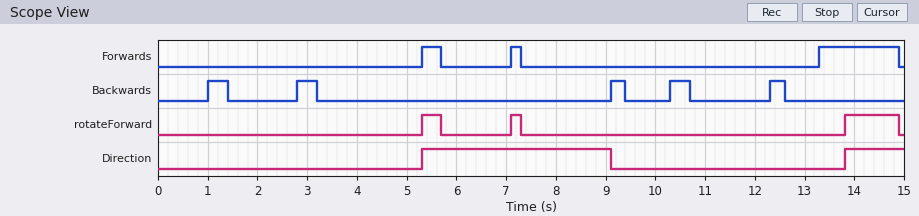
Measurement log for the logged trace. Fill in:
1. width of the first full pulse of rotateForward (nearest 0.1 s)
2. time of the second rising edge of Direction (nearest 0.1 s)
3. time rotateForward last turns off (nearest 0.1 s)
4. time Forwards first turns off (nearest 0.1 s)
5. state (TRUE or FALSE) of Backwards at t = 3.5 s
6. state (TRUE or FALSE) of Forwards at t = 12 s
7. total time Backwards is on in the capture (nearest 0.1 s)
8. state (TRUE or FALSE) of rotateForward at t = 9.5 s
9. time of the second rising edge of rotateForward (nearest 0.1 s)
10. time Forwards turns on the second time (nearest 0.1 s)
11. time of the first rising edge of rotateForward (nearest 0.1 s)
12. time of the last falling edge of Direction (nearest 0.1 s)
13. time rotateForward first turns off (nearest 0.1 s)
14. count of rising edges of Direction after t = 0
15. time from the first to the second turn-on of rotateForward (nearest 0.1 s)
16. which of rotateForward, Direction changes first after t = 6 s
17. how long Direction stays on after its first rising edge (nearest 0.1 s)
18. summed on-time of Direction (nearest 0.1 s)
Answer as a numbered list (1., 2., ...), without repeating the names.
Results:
1. 0.4 s
2. 13.8 s
3. 14.9 s
4. 5.7 s
5. FALSE
6. FALSE
7. 1.8 s
8. FALSE
9. 7.1 s
10. 7.1 s
11. 5.3 s
12. 9.1 s
13. 5.7 s
14. 2
15. 1.8 s
16. rotateForward
17. 3.8 s
18. 5.0 s
